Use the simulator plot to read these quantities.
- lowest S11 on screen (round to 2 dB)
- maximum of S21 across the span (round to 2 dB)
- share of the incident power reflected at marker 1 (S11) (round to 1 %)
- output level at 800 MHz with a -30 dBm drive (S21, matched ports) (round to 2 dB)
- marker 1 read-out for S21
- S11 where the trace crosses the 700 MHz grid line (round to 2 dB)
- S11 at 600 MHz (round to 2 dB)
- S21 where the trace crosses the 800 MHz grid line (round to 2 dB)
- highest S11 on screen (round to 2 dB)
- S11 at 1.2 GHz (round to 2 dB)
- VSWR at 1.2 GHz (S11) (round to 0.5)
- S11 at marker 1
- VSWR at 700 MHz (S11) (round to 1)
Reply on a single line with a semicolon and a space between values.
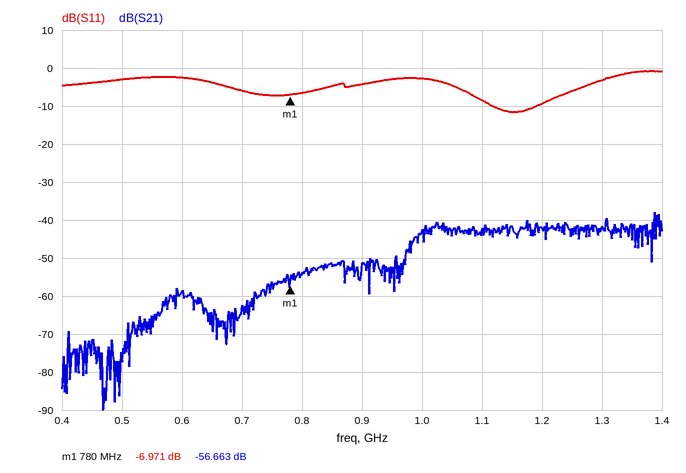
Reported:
-12 dB; -38 dB; 20 %; -84 dBm; -56.663 dB; -6 dB; -2 dB; -54 dB; 0 dB; -10 dB; 2.0; -6.971 dB; 3
